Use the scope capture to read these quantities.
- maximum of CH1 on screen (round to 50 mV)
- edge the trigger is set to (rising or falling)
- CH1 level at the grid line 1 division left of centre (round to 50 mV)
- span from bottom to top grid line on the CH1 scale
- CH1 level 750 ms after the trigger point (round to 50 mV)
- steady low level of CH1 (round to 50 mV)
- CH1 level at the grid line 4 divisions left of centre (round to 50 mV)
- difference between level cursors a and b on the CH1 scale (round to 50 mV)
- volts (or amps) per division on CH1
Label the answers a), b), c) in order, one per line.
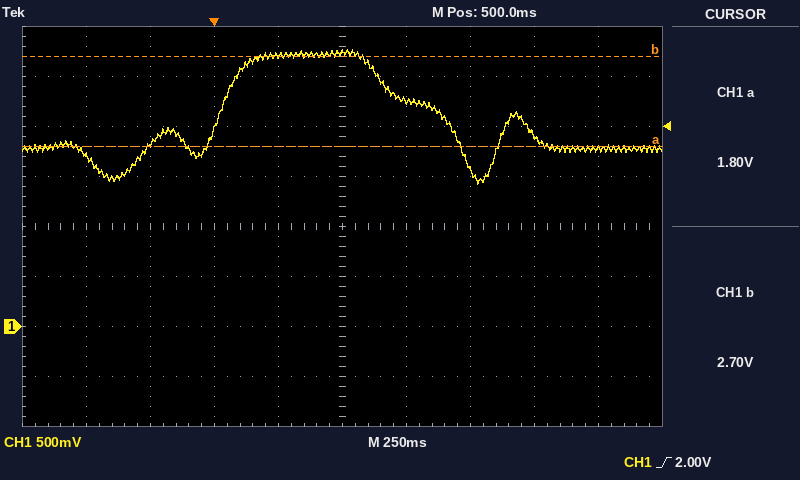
a) 2.75 V
b) rising
c) 2.70 V
d) 4 V
e) 2.25 V
f) 1.80 V
g) 1.70 V
h) 900 mV
i) 500 mV
